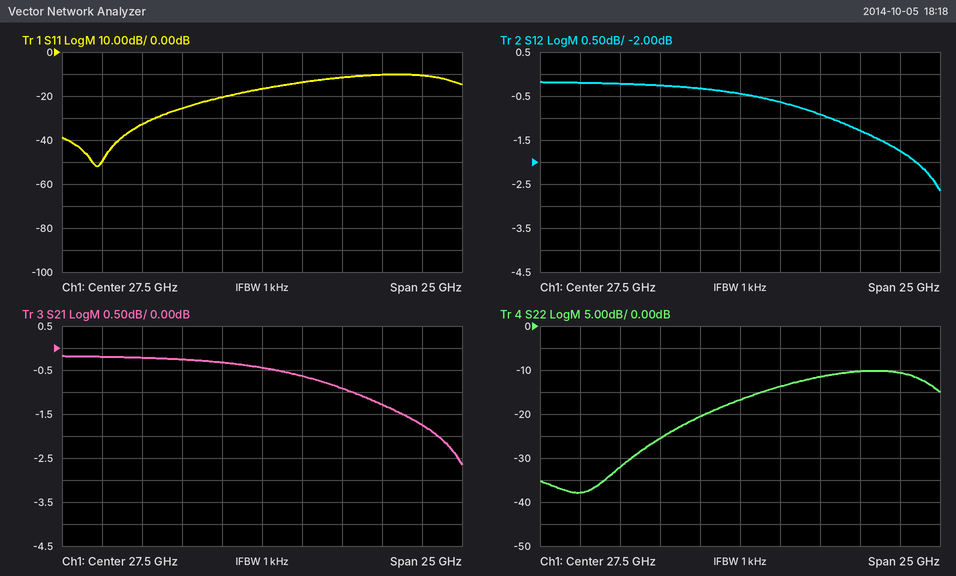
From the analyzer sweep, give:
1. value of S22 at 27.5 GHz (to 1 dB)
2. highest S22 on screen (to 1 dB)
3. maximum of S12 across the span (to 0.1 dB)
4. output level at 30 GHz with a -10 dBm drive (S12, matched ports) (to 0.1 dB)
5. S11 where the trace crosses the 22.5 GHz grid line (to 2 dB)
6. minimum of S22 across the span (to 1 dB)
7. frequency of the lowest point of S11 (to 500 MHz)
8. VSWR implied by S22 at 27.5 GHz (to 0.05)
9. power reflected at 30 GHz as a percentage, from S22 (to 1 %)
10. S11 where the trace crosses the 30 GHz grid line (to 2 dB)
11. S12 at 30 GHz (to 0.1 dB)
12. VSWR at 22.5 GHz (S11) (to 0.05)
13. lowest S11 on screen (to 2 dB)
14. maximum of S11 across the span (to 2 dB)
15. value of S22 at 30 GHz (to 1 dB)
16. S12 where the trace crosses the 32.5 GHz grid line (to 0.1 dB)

-17 dB
-10 dB
-0.2 dB
-10.6 dBm
-26 dB
-38 dB
17.0 GHz
1.35
4 %
-14 dB
-0.6 dB
1.10
-52 dB
-10 dB
-14 dB
-0.9 dB
